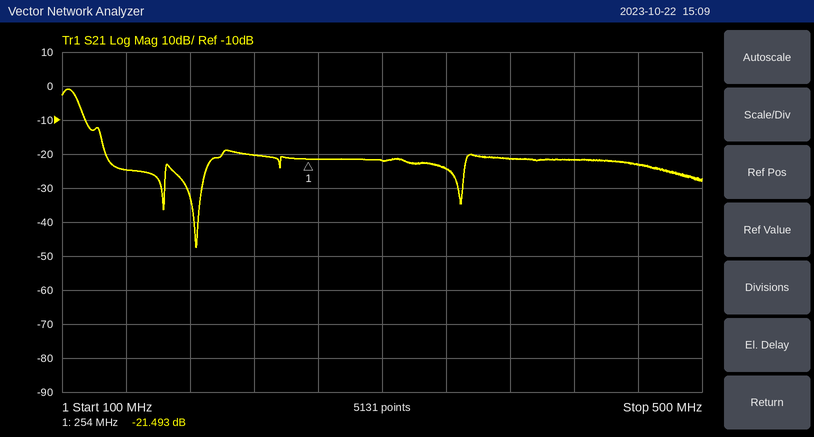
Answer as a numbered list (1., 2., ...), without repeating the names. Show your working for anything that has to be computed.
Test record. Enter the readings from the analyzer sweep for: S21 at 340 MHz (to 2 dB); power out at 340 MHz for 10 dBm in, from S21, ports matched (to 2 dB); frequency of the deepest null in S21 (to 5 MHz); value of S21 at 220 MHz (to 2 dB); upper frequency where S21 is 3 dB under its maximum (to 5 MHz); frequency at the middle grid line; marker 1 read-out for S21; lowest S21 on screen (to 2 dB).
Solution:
1. -24 dB
2. 10 dBm + (-24 dB) = -14 dBm
3. 185 MHz
4. -20 dB
5. 110 MHz
6. 300 MHz
7. -21.493 dB
8. -48 dB
